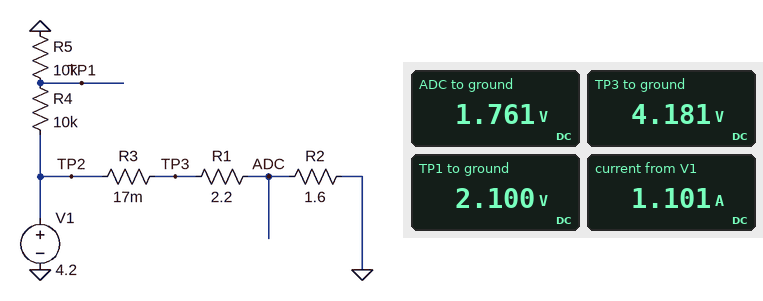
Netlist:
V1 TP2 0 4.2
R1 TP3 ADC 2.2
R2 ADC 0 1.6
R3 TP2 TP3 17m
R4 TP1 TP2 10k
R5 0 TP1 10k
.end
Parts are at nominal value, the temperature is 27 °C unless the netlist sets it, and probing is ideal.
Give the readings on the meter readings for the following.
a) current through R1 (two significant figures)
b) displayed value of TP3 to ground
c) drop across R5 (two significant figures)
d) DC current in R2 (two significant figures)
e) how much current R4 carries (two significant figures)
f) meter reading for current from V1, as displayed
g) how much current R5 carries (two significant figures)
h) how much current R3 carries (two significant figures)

1.1 A
4.181 V
2.1 V
1.1 A
210 µA
1.101 A
210 µA
1.1 A
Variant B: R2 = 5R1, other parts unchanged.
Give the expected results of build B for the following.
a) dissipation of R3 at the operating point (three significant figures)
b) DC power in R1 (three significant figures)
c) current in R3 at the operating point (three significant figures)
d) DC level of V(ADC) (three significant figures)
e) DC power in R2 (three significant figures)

5.60 mW
725 mW
574 mA
2.93 V
1.68 W
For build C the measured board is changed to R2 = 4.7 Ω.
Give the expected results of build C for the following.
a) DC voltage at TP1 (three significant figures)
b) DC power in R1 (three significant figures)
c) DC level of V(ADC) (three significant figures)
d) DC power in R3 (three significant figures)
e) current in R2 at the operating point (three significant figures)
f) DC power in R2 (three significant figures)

2.10 V
811 mW
2.85 V
6.27 mW
607 mA
1.73 W
